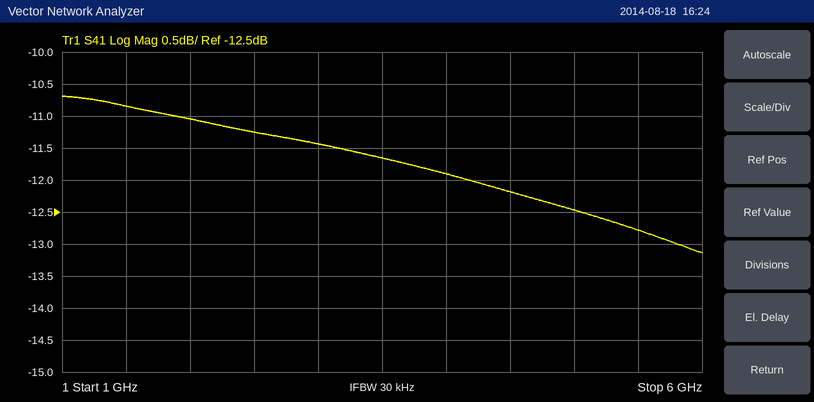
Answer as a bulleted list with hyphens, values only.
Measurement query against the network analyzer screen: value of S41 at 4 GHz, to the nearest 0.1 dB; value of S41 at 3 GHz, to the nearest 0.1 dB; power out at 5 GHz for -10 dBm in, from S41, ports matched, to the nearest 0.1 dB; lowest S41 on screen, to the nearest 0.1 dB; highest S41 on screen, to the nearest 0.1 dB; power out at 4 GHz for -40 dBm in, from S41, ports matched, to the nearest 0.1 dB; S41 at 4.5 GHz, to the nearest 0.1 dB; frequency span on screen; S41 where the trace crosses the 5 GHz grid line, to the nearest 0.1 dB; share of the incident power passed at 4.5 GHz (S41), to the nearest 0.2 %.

- -11.9 dB
- -11.4 dB
- -22.5 dBm
- -13.1 dB
- -10.7 dB
- -51.9 dBm
- -12.2 dB
- 5 GHz
- -12.5 dB
- 6.0 %
